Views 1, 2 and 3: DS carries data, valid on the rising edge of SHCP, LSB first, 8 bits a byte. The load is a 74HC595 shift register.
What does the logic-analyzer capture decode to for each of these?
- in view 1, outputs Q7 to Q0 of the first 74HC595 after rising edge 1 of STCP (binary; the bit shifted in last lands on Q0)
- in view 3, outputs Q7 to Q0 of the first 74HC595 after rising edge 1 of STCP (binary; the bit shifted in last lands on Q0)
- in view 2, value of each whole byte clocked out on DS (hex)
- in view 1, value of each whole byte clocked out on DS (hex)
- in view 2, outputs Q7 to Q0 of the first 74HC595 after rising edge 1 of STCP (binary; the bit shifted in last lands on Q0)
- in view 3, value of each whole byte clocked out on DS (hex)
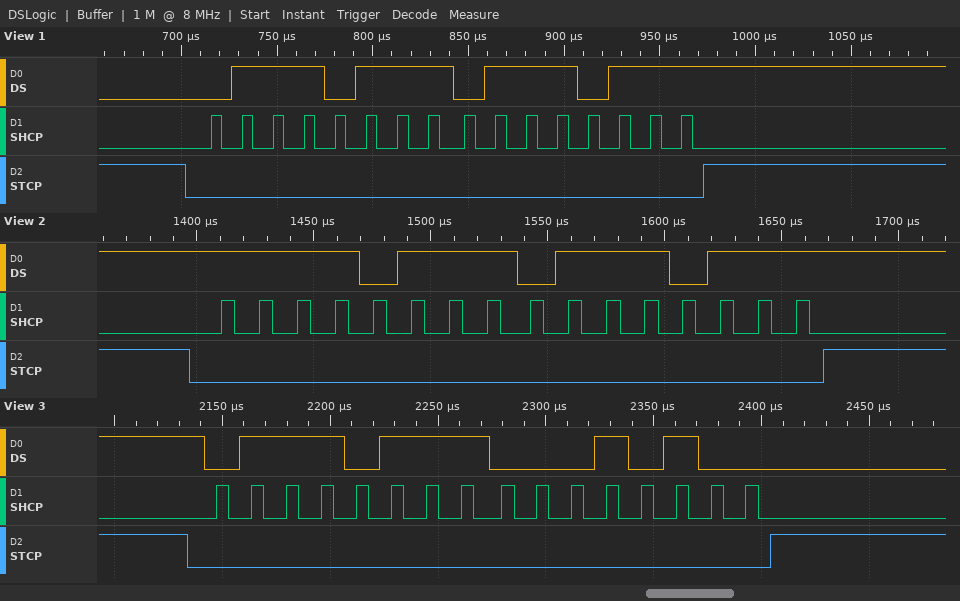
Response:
01110111
00010100
EF EE
EE EE
01110111
EE 28
